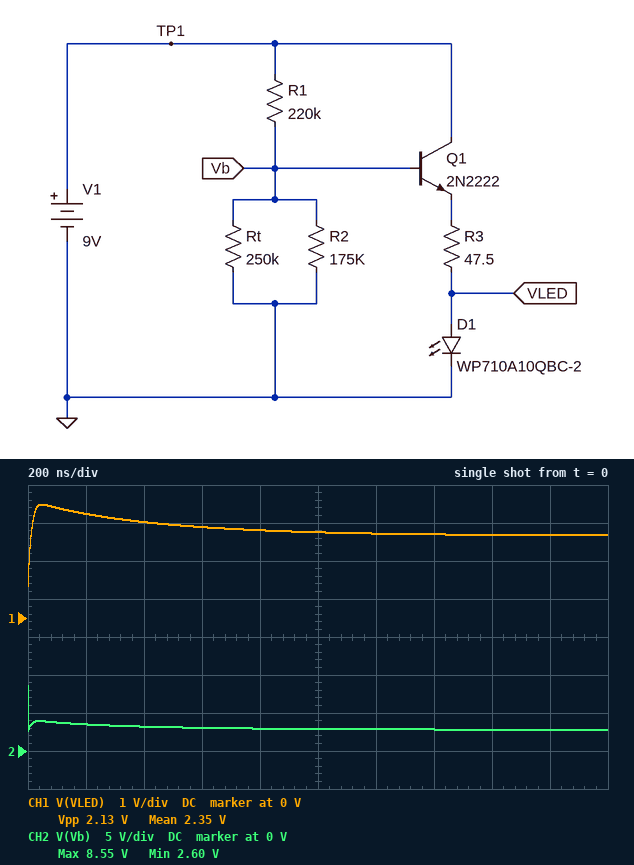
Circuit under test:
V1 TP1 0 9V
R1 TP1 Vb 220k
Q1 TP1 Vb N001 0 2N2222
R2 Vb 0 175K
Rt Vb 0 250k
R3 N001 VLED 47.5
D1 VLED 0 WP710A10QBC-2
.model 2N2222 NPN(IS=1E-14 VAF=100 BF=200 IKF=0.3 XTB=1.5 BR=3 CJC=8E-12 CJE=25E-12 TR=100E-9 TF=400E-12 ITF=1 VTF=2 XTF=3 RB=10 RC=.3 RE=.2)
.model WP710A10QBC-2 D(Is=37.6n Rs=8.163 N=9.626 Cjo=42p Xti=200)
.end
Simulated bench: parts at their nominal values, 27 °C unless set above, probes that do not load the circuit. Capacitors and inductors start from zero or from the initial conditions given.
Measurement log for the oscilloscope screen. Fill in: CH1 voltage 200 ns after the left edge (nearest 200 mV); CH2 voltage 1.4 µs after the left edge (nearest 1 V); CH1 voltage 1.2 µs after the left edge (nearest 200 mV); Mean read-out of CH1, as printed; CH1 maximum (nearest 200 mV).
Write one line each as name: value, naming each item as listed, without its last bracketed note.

CH1 voltage 200 ns after the left edge: 2.8 V
CH2 voltage 1.4 µs after the left edge: 3 V
CH1 voltage 1.2 µs after the left edge: 2.2 V
Mean read-out of CH1, as printed: 2.35 V
CH1 maximum: 3.0 V
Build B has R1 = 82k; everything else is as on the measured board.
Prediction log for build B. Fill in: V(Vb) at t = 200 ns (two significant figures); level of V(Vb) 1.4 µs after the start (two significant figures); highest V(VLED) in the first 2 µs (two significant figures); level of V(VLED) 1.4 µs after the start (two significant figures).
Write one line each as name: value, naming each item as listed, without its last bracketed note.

V(Vb) at t = 200 ns: 4.0 V
level of V(Vb) 1.4 µs after the start: 3.9 V
highest V(VLED) in the first 2 µs: 3.1 V
level of V(VLED) 1.4 µs after the start: 3.0 V
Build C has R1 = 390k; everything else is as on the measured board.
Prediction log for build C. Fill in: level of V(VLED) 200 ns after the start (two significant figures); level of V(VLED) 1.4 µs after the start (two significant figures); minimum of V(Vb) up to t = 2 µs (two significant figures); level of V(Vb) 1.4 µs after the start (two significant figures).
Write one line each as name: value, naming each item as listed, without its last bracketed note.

level of V(VLED) 200 ns after the start: 2.6 V
level of V(VLED) 1.4 µs after the start: 1.7 V
minimum of V(Vb) up to t = 2 µs: 2.0 V
level of V(Vb) 1.4 µs after the start: 2.2 V
